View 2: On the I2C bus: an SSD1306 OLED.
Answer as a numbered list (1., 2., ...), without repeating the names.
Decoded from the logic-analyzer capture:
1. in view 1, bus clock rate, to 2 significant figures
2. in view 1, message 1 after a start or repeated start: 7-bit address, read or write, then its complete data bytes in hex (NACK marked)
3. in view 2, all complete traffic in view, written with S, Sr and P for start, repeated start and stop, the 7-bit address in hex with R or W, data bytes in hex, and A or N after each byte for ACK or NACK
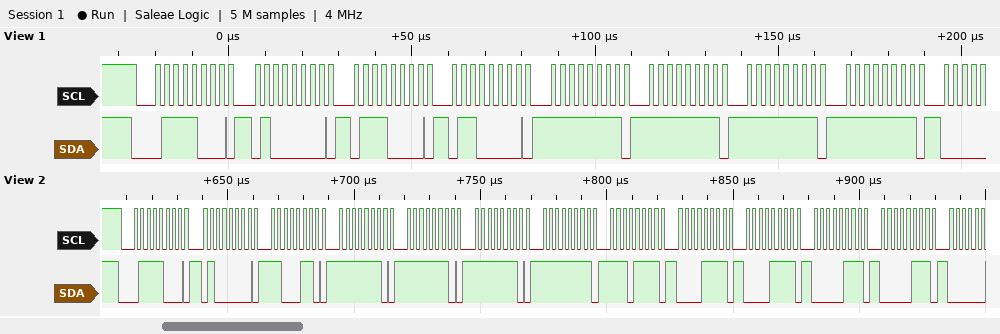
1. 400 kHz
2. 0x3C write: 40 70 60 FF FF FF FF
3. S 3CW A 40 A C6 A FE A FE A FE A FF A EF A 0F A 0F A 07 A 07 A
